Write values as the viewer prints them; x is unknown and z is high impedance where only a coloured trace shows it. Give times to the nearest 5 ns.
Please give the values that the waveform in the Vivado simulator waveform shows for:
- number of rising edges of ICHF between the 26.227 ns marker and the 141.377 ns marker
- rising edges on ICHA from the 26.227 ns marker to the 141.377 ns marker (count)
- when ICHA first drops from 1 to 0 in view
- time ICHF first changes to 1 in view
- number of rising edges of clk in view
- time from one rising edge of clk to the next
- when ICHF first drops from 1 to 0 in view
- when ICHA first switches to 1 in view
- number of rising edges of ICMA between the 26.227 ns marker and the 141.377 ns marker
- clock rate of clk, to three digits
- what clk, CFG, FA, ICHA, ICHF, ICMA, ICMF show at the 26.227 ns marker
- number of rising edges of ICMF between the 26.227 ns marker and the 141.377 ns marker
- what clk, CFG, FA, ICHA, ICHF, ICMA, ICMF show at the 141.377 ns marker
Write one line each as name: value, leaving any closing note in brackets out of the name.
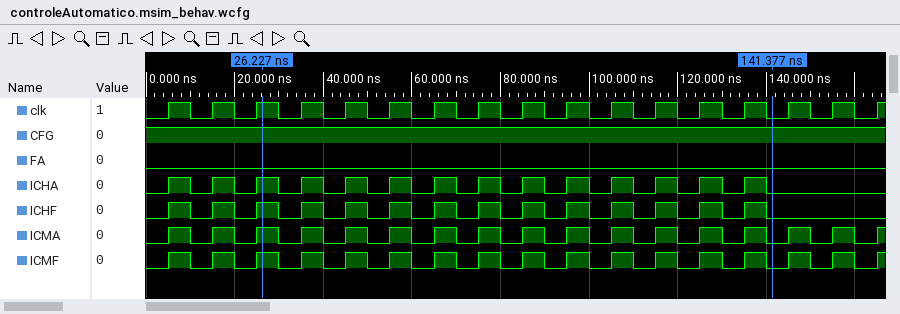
number of rising edges of ICHF between the 26.227 ns marker and the 141.377 ns marker: 11
rising edges on ICHA from the 26.227 ns marker to the 141.377 ns marker: 11
when ICHA first drops from 1 to 0 in view: 10 ns
time ICHF first changes to 1 in view: 5 ns
number of rising edges of clk in view: 17
time from one rising edge of clk to the next: 10 ns
when ICHF first drops from 1 to 0 in view: 10 ns
when ICHA first switches to 1 in view: 5 ns
number of rising edges of ICMA between the 26.227 ns marker and the 141.377 ns marker: 11
clock rate of clk, to three digits: 100 MHz
what clk, CFG, FA, ICHA, ICHF, ICMA, ICMF show at the 26.227 ns marker: clk=1, CFG=1, FA=0, ICHA=1, ICHF=1, ICMA=1, ICMF=1
number of rising edges of ICMF between the 26.227 ns marker and the 141.377 ns marker: 11
what clk, CFG, FA, ICHA, ICHF, ICMA, ICMF show at the 141.377 ns marker: clk=0, CFG=1, FA=0, ICHA=0, ICHF=0, ICMA=0, ICMF=0
